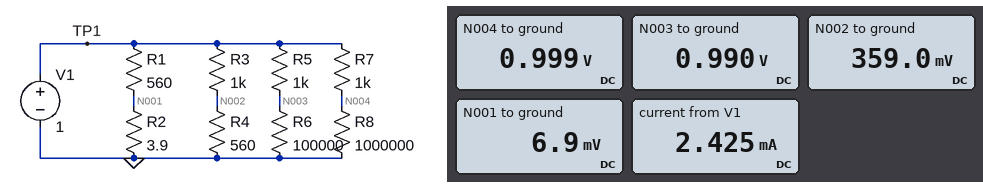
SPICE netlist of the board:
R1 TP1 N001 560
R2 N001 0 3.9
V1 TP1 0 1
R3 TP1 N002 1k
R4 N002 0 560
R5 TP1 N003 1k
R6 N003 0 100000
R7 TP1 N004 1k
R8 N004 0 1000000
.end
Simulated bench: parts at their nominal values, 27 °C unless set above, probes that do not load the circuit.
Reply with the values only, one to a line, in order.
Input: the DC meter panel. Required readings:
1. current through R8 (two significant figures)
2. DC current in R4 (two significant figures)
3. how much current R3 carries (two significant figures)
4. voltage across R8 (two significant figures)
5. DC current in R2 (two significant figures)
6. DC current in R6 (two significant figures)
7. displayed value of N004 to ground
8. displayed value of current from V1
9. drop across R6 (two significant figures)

1.0 µA
640 µA
640 µA
1.0 V
1.8 mA
9.9 µA
0.999 V
2.425 mA
990 mV
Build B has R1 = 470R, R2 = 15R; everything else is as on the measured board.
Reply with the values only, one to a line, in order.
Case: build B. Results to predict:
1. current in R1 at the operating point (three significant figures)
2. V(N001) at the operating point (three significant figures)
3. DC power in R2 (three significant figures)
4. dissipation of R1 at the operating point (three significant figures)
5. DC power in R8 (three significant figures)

2.06 mA
30.9 mV
63.8 µW
2.00 mW
998 nW
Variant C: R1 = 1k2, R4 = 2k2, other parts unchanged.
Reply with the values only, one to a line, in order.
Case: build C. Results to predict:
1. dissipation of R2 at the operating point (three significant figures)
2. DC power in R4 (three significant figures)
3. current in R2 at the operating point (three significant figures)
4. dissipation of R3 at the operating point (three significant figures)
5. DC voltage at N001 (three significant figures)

2.69 µW
215 µW
831 µA
97.7 µW
3.24 mV
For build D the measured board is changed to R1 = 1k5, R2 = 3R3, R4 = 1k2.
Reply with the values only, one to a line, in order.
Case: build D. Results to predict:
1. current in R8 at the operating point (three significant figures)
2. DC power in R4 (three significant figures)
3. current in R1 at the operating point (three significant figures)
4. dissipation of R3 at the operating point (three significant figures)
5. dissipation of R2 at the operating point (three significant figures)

999 nA
248 µW
665 µA
207 µW
1.46 µW
